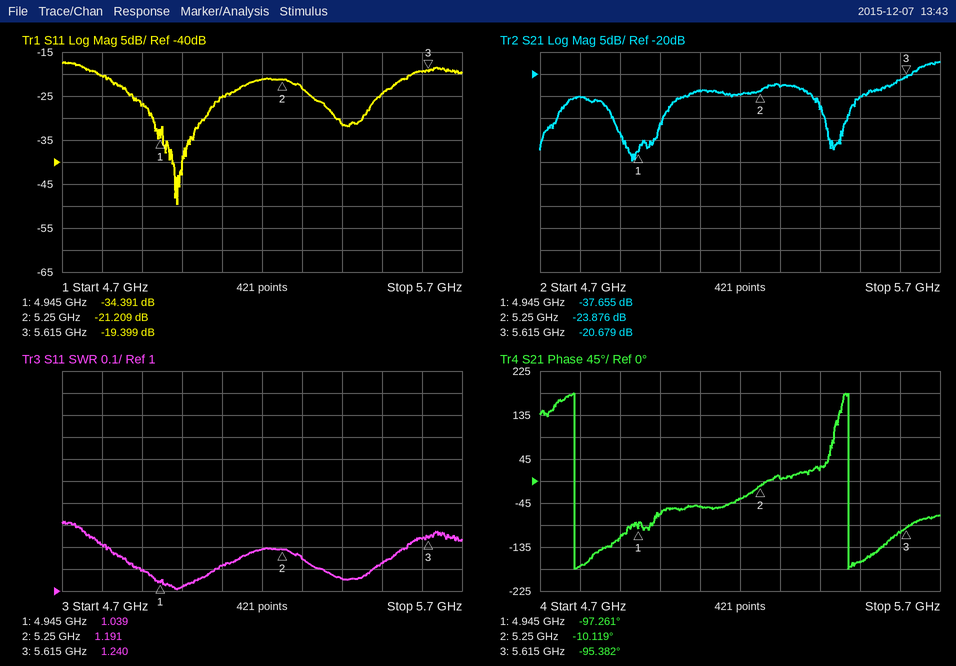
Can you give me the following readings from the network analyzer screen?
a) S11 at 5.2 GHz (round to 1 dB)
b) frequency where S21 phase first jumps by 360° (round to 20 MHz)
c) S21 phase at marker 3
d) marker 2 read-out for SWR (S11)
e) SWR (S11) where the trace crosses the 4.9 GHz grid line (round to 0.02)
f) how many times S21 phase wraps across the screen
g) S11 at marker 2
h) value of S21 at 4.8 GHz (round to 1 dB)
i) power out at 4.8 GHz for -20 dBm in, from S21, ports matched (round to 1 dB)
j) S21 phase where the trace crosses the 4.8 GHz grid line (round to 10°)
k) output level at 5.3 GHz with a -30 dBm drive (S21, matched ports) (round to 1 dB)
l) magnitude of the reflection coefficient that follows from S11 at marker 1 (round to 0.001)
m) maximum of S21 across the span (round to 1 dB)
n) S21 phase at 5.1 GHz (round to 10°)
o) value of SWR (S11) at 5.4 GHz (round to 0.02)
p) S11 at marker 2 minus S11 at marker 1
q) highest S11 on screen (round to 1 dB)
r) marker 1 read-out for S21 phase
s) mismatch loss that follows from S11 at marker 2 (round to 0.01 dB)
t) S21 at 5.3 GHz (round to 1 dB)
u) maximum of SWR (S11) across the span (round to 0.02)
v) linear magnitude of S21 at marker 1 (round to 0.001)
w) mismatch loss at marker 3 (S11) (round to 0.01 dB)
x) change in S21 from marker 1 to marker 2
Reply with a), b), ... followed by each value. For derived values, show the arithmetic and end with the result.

a) -21 dB
b) 4.78 GHz
c) -95.382°
d) 1.191
e) 1.10
f) 2
g) -21.209 dB
h) -25 dB
i) -20 dBm + (-25 dB) = -45 dBm
j) -170°
k) -30 dBm + (-23 dB) = -53 dBm
l) 10^(-34.391/20) ≈ 0.019
m) -17 dB
n) -50°
o) 1.06
p) -21.209 − (-34.391) = 13.182 dB
q) -17 dB
r) -97.261°
s) −10 log10(1 − 10^(-21.209/10)) ≈ 0.03 dB
t) -23 dB
u) 1.32
v) 10^(-37.655/20) ≈ 0.013
w) −10 log10(1 − 10^(-19.399/10)) ≈ 0.05 dB
x) -23.876 − (-37.655) = 13.779 dB
